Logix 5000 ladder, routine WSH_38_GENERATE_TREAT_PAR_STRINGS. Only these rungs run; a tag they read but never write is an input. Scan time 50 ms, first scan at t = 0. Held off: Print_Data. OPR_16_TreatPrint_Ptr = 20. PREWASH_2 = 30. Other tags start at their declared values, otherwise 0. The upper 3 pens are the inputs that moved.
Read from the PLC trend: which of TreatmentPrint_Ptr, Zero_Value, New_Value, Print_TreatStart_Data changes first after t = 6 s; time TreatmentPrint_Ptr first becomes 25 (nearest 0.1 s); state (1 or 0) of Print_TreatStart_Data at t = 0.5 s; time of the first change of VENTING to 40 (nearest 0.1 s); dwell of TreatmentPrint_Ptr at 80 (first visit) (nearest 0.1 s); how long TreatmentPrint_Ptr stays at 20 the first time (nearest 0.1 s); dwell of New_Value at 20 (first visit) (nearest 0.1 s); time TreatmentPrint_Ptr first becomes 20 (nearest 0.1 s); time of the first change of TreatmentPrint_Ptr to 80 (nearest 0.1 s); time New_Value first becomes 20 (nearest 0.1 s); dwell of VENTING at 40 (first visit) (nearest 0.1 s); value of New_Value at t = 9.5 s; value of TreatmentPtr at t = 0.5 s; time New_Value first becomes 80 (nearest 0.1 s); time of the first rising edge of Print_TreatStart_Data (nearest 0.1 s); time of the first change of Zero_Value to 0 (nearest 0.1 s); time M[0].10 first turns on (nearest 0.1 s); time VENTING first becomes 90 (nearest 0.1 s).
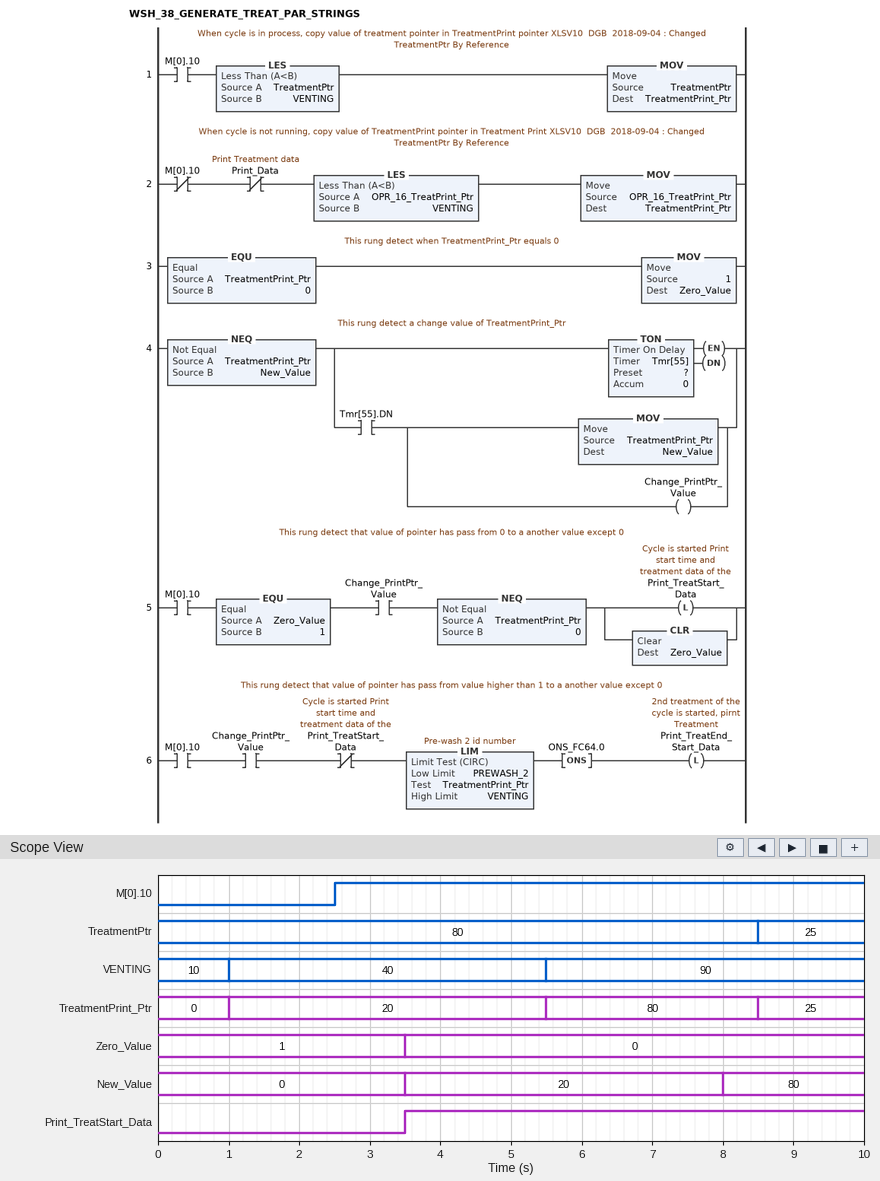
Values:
New_Value
8.5 s
0
1.0 s
3.0 s
4.5 s
4.5 s
1.0 s
5.5 s
3.5 s
4.5 s
80
80
8.0 s
3.5 s
3.5 s
2.5 s
5.5 s
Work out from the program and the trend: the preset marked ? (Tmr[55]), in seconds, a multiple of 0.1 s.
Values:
2.5 s
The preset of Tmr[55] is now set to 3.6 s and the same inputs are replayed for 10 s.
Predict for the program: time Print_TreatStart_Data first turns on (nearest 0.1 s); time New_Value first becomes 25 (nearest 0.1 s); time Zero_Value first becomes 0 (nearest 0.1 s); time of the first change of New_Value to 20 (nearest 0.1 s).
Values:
4.6 s
9.1 s
4.6 s
4.6 s
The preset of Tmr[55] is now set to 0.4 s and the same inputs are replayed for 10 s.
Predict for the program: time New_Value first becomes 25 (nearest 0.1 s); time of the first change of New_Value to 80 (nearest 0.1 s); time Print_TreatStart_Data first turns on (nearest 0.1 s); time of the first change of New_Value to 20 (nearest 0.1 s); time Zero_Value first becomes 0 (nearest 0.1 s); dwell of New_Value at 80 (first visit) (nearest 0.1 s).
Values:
8.9 s
5.9 s
5.9 s
1.4 s
5.9 s
3.0 s
